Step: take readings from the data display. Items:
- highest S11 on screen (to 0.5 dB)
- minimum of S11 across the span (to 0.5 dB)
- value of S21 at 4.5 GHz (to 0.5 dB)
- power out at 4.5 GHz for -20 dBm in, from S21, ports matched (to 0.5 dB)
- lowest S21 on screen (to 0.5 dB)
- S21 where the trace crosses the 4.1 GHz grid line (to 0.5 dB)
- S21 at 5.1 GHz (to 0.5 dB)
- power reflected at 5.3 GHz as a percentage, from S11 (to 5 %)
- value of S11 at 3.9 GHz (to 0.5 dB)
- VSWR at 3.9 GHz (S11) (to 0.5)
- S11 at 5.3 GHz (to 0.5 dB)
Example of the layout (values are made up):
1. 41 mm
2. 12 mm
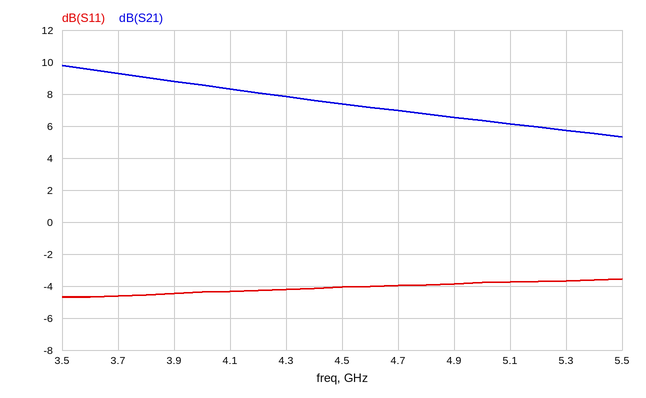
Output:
1. -3.5 dB
2. -4.5 dB
3. 7.5 dB
4. -12.5 dBm
5. 5.5 dB
6. 8.5 dB
7. 6.0 dB
8. 45 %
9. -4.5 dB
10. 4.0
11. -3.5 dB
